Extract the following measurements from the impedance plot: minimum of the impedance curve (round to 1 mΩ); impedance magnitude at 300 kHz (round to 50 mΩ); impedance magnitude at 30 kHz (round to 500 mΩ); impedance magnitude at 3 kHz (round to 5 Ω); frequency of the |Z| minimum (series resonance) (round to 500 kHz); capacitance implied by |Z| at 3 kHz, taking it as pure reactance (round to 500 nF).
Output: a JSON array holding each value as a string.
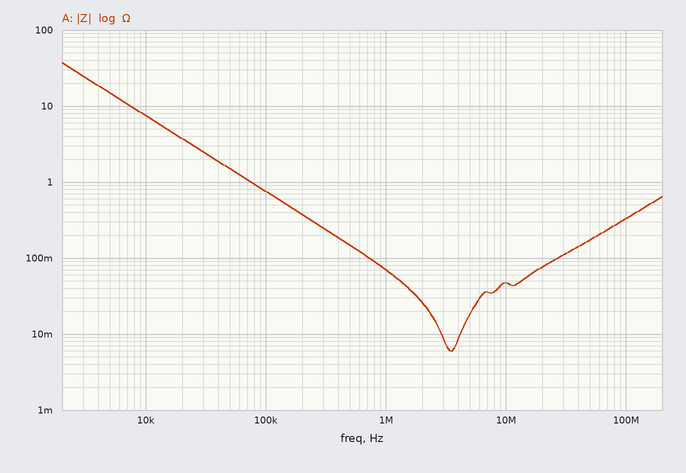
["6 mΩ", "250 mΩ", "2.5 Ω", "25 Ω", "3.5 MHz", "2.0 µF"]
